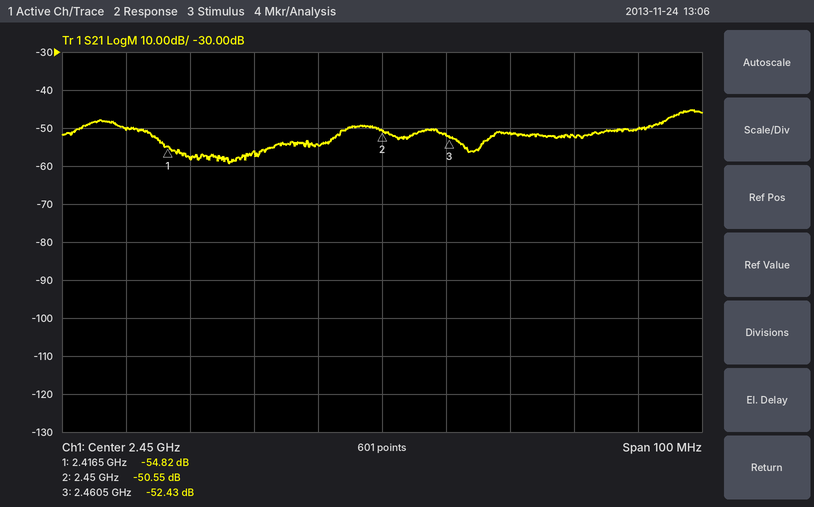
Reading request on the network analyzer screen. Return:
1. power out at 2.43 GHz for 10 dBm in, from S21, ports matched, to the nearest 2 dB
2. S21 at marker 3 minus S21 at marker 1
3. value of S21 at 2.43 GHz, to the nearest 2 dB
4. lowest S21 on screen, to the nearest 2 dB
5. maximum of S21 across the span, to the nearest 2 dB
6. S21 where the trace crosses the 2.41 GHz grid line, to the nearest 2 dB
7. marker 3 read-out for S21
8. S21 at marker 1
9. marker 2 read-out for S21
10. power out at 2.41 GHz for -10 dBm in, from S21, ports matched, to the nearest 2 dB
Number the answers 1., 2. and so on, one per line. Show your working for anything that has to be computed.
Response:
1. 10 dBm + (-56 dB) = -46 dBm
2. -52.43 − (-54.82) = 2.39 dB
3. -56 dB
4. -60 dB
5. -46 dB
6. -50 dB
7. -52.43 dB
8. -54.82 dB
9. -50.55 dB
10. -10 dBm + (-50 dB) = -60 dBm
